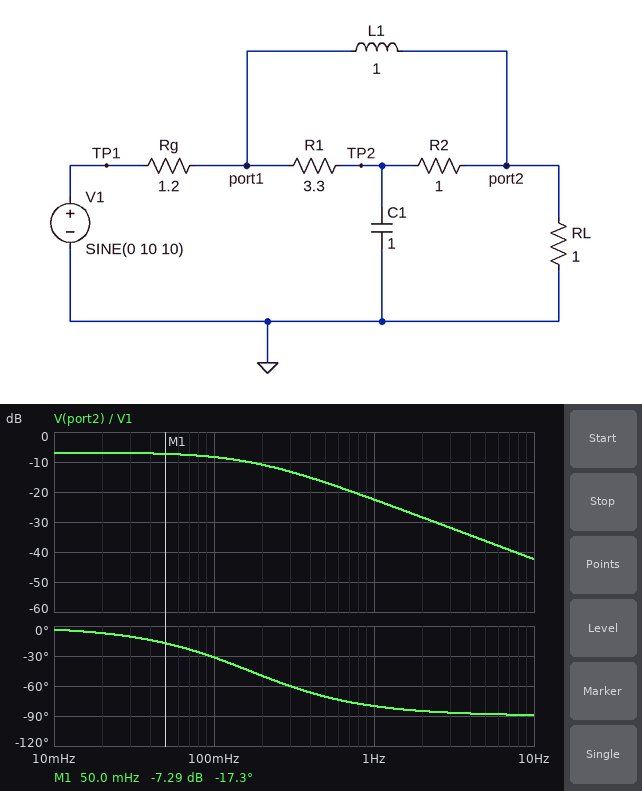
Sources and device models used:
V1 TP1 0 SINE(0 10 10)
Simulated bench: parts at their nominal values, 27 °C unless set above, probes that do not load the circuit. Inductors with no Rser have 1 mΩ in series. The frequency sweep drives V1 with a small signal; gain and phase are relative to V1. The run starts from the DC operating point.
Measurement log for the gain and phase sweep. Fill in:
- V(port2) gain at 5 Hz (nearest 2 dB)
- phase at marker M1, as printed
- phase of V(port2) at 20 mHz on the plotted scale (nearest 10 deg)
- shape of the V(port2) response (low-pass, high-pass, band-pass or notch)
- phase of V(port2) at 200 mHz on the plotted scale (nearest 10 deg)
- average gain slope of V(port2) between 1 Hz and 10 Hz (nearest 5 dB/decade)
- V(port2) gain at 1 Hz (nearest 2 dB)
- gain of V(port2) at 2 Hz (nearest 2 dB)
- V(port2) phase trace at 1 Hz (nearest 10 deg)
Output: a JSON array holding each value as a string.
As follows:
["-36 dB", "-17.3 deg", "-10 deg", "low-pass", "-50 deg", "-20 dB/decade", "-22 dB", "-28 dB", "-80 deg"]
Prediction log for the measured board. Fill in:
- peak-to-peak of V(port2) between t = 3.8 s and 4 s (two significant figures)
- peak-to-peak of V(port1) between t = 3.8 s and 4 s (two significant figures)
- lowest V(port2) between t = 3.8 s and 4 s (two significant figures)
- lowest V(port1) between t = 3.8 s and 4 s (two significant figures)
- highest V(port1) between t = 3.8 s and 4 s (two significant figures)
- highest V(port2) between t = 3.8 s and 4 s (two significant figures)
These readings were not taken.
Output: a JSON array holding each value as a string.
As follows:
["150 mV", "15 V", "-75 mV", "-7.3 V", "7.3 V", "78 mV"]
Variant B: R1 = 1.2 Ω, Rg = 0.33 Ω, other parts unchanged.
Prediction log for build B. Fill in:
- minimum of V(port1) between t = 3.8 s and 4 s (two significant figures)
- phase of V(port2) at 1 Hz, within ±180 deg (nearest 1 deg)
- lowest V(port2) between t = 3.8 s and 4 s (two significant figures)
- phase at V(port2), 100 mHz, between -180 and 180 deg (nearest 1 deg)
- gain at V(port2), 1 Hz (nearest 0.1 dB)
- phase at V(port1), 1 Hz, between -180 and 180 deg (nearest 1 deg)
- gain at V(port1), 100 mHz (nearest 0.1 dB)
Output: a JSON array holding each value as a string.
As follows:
["-7.8 V", "-82 deg", "-110 mV", "-33 deg", "-18.9 dB", "1 deg", "-2.5 dB"]
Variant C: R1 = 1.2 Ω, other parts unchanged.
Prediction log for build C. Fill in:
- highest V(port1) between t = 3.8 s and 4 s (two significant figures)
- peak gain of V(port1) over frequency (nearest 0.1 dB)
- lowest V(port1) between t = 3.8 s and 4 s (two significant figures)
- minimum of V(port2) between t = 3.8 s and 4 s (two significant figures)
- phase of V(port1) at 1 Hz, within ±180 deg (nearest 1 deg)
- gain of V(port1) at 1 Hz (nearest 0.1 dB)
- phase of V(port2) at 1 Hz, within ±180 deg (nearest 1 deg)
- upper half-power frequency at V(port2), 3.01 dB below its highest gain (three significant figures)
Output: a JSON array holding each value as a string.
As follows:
["5.0 V", "-6.0 dB", "-5.0 V", "-72 mV", "2 deg", "-6.1 dB", "-81 deg", "159 mHz"]
